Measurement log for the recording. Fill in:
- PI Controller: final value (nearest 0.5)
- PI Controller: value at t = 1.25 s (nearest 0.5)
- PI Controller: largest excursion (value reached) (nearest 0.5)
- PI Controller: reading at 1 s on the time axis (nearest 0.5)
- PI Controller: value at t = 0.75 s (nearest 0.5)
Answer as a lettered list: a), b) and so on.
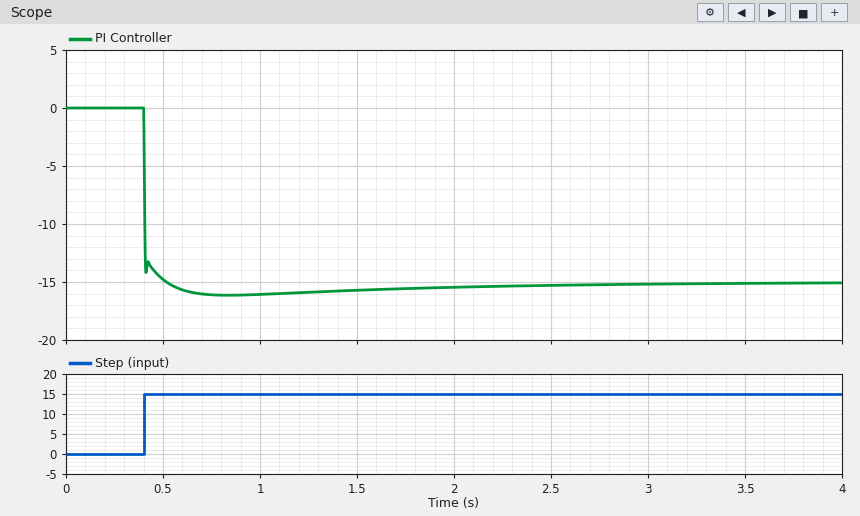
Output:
a) -15.0
b) -16.0
c) -16.0
d) -16.0
e) -16.0
